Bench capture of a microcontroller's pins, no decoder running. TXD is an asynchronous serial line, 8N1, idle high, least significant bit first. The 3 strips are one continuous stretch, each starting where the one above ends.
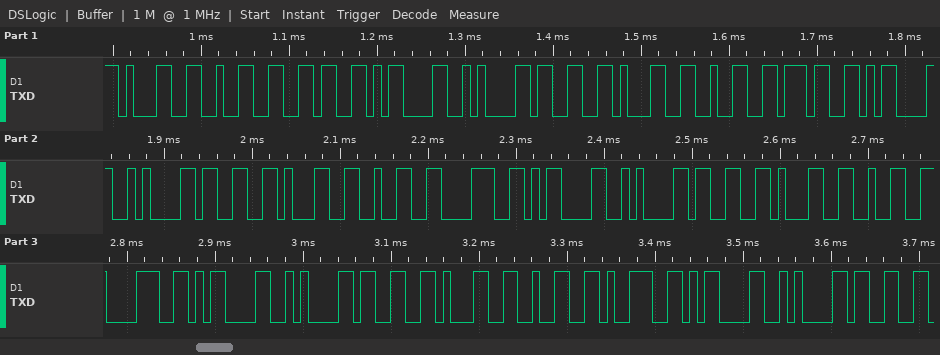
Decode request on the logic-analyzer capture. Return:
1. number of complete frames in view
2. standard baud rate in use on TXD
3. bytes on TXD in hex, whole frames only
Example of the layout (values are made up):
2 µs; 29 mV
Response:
30; 115200 baud; 31 32 36 0D 0A 33 31 32 37 0D 0A 33 31 32 38 0D 0A 33 31 32 38 0D 0A 33 31 32 39 0D 0A 33
